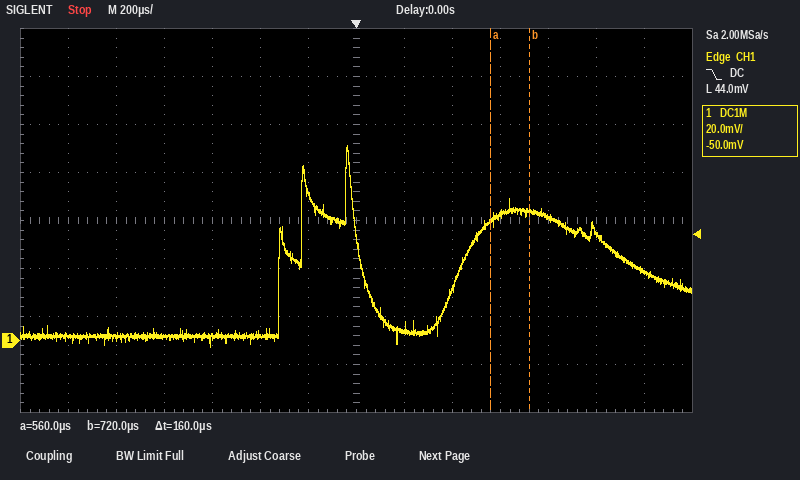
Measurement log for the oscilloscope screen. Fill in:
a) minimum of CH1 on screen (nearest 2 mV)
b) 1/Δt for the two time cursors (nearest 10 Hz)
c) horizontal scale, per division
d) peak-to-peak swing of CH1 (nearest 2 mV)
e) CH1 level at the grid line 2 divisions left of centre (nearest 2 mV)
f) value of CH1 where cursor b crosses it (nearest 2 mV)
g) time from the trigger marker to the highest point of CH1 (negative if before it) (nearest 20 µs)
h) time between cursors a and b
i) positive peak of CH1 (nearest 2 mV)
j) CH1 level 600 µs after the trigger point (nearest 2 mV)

-2 mV
6.25 kHz
200 µs
84 mV
2 mV
54 mV
-40 µs
160 µs
82 mV
52 mV
